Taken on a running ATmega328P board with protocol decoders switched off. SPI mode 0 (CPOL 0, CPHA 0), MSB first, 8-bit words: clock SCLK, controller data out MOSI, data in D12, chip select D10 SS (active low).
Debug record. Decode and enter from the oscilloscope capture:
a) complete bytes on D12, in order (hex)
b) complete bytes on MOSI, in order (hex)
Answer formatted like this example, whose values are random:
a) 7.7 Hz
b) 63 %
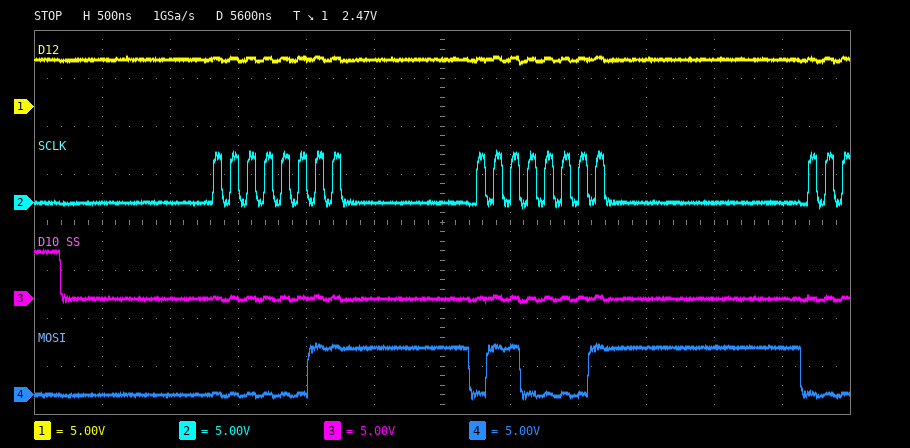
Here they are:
a) FF FF
b) 03 61
